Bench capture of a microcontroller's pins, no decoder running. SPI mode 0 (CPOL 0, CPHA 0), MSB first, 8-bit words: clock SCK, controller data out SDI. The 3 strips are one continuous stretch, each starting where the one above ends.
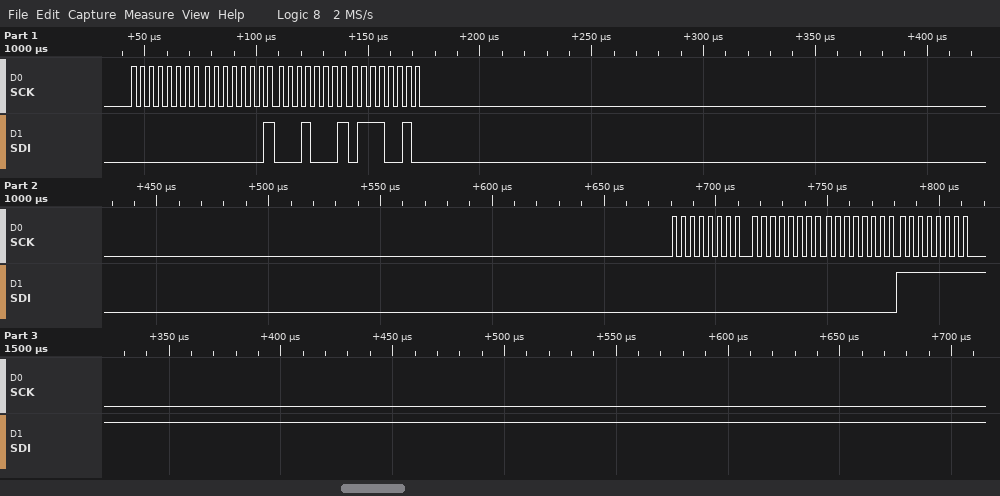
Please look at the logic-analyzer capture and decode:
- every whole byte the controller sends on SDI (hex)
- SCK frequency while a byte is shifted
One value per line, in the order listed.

00 01 11 72 00 00 00 FF
250 kHz
